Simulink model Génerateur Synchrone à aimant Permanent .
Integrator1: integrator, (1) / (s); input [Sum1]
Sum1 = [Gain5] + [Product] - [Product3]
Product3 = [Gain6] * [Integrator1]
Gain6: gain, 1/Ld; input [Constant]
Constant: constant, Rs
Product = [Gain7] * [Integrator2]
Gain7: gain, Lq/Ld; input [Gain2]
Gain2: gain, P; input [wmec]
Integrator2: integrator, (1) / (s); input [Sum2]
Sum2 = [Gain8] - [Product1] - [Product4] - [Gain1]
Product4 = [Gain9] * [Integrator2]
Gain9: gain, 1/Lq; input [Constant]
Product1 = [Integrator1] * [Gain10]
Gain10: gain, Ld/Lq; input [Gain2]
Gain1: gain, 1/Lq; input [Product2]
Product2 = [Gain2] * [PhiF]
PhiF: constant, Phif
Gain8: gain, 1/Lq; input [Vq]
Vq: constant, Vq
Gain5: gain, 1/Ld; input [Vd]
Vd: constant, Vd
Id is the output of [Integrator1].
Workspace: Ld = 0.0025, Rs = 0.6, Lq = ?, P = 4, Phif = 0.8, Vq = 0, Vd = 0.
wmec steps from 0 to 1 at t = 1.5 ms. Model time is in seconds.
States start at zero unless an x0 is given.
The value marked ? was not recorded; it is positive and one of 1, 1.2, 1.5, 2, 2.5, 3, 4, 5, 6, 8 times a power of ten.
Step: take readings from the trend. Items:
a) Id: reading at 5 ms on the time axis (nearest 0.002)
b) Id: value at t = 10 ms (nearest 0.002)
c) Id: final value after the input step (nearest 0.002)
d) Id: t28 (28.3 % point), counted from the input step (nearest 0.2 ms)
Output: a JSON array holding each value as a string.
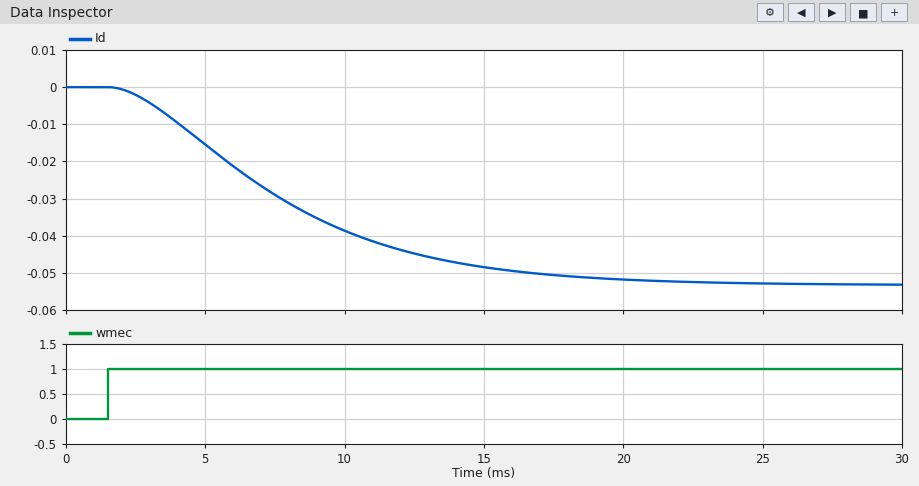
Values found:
["-0.016", "-0.038", "-0.054", "3.4 ms"]
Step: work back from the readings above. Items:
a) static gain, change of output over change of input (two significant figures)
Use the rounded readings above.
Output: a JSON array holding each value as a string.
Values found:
["-0.054"]
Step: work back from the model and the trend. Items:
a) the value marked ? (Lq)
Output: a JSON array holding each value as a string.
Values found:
["0.0015"]
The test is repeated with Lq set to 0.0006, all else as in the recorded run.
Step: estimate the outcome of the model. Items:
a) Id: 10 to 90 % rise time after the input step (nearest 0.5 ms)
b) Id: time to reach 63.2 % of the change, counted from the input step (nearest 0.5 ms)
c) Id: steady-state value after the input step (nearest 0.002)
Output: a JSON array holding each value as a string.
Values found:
["9.5 ms", "5.5 ms", "-0.022"]
